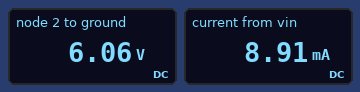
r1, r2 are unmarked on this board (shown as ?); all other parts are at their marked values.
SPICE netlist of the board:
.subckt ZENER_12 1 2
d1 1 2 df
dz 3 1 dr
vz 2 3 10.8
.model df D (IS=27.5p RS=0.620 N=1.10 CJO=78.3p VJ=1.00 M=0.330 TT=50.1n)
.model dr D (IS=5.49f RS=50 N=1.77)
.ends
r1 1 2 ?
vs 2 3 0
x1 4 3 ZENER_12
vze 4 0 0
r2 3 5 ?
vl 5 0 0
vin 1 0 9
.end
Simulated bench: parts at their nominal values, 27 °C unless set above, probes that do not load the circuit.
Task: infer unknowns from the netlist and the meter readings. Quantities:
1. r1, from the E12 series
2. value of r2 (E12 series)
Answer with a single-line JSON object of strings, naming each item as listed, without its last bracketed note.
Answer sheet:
{"r1, from the E12 series": "330 Ω", "value of r2": "680 Ω"}
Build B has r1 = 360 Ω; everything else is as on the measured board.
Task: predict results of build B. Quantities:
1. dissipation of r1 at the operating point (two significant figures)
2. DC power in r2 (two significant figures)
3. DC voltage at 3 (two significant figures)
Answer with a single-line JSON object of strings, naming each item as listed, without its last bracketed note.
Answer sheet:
{"dissipation of r1 at the operating point": "27 mW", "DC power in r2": "51 mW", "DC voltage at 3": "5.9 V"}
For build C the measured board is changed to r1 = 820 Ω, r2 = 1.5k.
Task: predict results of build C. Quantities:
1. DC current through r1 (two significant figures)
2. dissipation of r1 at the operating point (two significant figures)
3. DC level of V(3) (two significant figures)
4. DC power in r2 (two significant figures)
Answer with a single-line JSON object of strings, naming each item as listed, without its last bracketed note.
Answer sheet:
{"DC current through r1": "3.9 mA", "dissipation of r1 at the operating point": "12 mW", "DC level of V(3)": "5.8 V", "DC power in r2": "23 mW"}
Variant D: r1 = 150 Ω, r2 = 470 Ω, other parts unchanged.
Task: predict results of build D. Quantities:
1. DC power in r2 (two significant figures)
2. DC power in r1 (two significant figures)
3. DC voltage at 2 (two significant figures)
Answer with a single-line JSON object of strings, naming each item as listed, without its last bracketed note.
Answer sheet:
{"DC power in r2": "99 mW", "DC power in r1": "32 mW", "DC voltage at 2": "6.8 V"}
